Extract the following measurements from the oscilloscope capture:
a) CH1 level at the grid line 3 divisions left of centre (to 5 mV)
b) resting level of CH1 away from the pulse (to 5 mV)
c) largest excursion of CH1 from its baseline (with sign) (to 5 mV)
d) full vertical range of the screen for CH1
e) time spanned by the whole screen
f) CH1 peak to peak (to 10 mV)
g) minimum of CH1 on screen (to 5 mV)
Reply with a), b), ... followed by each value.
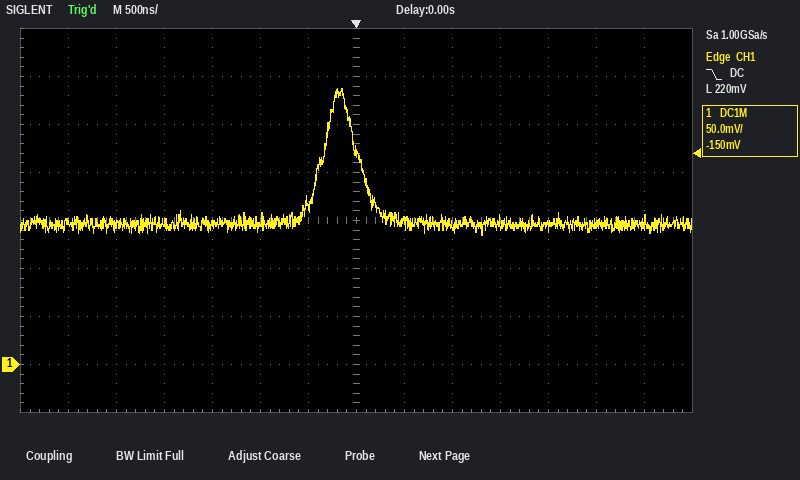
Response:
a) 145 mV
b) 145 mV
c) +140 mV
d) 400 mV
e) 7 µs
f) 150 mV
g) 135 mV
